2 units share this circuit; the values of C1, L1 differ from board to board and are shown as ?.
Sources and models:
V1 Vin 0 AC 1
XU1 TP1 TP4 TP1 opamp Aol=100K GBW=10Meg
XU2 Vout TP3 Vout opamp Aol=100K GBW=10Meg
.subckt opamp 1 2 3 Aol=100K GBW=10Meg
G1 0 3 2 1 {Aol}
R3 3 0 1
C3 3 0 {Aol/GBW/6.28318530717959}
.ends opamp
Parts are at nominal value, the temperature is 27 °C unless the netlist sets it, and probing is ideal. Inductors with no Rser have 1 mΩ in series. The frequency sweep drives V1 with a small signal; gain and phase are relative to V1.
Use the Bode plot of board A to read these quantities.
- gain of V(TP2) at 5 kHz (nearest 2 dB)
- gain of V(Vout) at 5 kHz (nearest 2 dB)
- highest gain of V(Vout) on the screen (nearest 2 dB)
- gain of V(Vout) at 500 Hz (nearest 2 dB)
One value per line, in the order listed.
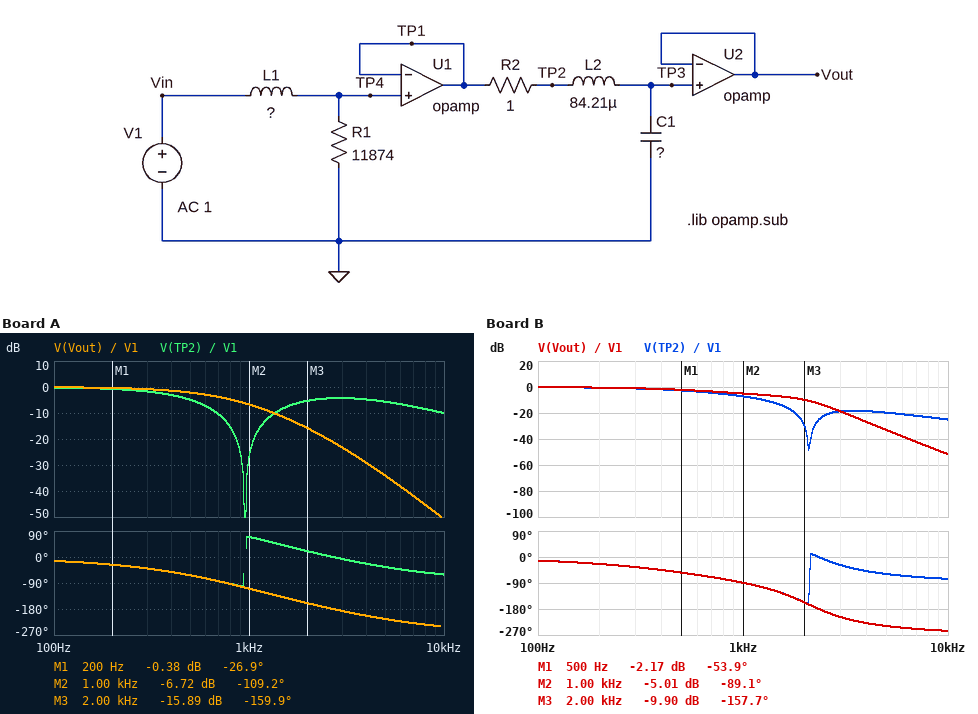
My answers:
-6 dB
-34 dB
0 dB
-2 dB
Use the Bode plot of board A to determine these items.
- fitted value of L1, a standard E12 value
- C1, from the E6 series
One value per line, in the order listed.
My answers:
560 mH
330 µF
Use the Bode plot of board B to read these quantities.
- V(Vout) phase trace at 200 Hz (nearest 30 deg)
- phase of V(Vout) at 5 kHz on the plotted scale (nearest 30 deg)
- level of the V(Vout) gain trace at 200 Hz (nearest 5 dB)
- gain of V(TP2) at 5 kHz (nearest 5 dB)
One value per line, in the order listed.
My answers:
-30 deg
-240 deg
0 dB
-20 dB
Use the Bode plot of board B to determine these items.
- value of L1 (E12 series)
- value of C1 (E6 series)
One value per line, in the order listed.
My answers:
3.3 H
68 µF
